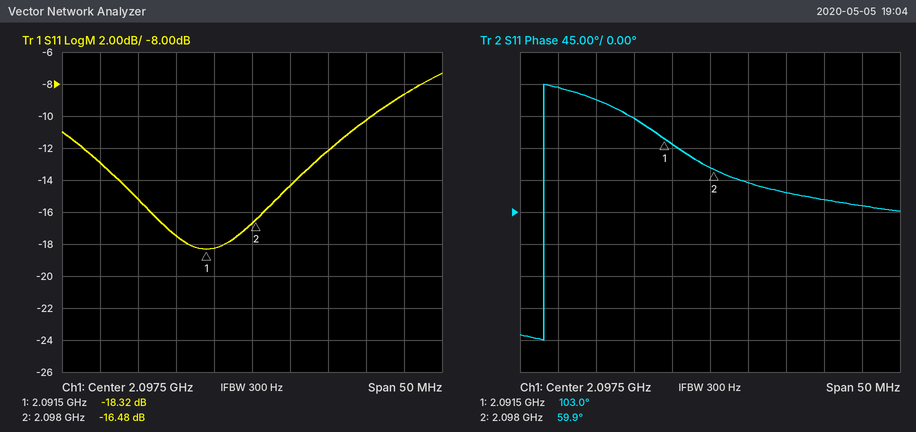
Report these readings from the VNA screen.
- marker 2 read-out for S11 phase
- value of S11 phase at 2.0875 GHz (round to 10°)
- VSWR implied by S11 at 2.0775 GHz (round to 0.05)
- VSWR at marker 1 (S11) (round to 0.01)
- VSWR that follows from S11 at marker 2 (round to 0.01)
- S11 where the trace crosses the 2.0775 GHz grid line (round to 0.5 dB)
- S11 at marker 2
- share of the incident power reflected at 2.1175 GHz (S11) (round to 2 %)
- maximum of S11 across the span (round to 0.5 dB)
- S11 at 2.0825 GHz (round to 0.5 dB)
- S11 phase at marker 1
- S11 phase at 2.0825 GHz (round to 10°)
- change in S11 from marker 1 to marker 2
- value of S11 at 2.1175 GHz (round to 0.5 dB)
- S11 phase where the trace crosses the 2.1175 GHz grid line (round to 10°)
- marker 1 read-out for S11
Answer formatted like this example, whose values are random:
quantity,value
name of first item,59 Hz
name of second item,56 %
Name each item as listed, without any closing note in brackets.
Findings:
quantity,value
marker 2 read-out for S11 phase,59.9°
value of S11 phase at 2.0875 GHz,130°
VSWR implied by S11 at 2.0775 GHz,1.60
VSWR at marker 1 (S11),1.28
VSWR that follows from S11 at marker 2,1.35
S11 where the trace crosses the 2.0775 GHz grid line,-13.0 dB
S11 at marker 2,-16.48 dB
share of the incident power reflected at 2.1175 GHz (S11),14 %
maximum of S11 across the span,-7.5 dB
S11 at 2.0825 GHz,-15.0 dB
S11 phase at marker 1,103.0°
S11 phase at 2.0825 GHz,160°
change in S11 from marker 1 to marker 2,1.84 dB
value of S11 at 2.1175 GHz,-8.5 dB
S11 phase where the trace crosses the 2.1175 GHz grid line,10°
marker 1 read-out for S11,-18.32 dB
